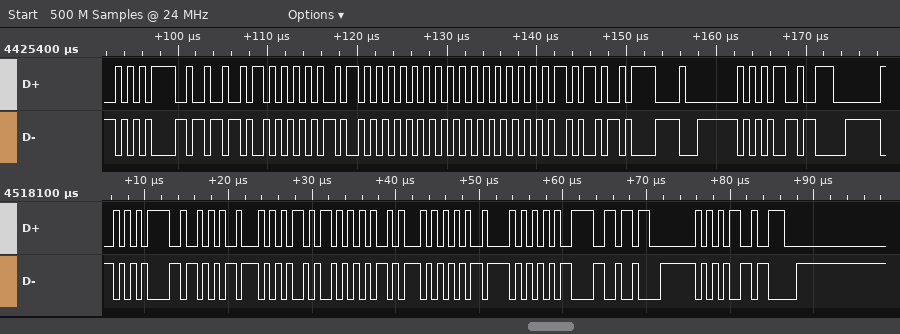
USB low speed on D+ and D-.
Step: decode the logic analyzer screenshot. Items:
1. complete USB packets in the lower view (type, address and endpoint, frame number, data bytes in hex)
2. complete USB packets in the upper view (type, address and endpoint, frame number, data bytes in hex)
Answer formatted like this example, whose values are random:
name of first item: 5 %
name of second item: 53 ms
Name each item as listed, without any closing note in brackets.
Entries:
complete USB packets in the lower view: DATA1 [ 20 03 42 00 61 00 72 00 ], ACK
complete USB packets in the upper view: DATA1 [ 12 01 10 01 00 00 00 08 ], ACK
